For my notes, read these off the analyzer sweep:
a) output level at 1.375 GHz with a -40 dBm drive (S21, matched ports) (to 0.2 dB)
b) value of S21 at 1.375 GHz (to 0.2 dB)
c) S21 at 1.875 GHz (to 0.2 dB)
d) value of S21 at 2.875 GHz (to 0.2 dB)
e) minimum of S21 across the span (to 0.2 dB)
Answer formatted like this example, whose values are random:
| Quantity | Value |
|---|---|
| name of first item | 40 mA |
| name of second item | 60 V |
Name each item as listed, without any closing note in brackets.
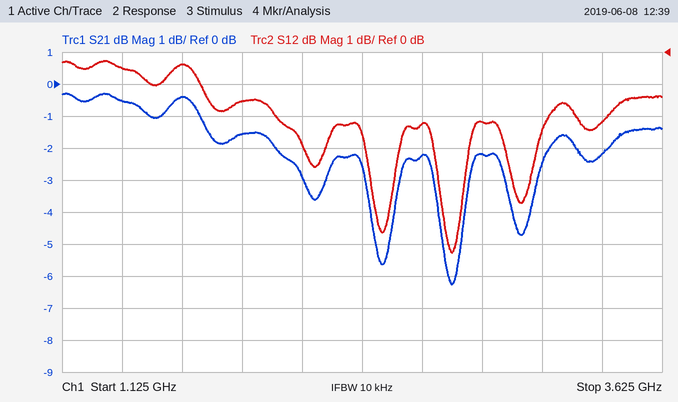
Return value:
| Quantity | Value |
|---|---|
| output level at 1.375 GHz with a -40 dBm drive (S21, matched ports) | -40.6 dBm |
| value of S21 at 1.375 GHz | -0.6 dB |
| S21 at 1.875 GHz | -1.6 dB |
| value of S21 at 2.875 GHz | -2.2 dB |
| minimum of S21 across the span | -6.2 dB |
